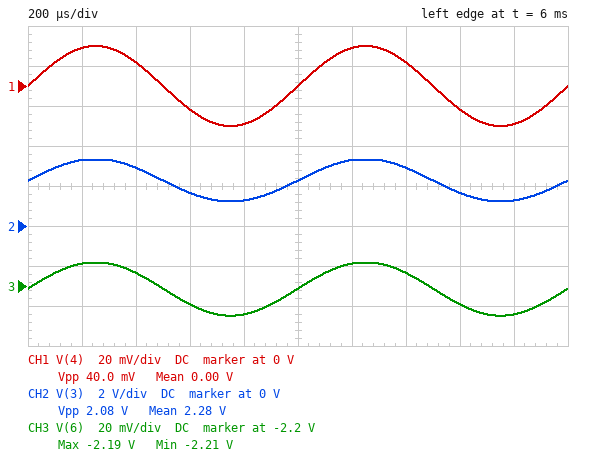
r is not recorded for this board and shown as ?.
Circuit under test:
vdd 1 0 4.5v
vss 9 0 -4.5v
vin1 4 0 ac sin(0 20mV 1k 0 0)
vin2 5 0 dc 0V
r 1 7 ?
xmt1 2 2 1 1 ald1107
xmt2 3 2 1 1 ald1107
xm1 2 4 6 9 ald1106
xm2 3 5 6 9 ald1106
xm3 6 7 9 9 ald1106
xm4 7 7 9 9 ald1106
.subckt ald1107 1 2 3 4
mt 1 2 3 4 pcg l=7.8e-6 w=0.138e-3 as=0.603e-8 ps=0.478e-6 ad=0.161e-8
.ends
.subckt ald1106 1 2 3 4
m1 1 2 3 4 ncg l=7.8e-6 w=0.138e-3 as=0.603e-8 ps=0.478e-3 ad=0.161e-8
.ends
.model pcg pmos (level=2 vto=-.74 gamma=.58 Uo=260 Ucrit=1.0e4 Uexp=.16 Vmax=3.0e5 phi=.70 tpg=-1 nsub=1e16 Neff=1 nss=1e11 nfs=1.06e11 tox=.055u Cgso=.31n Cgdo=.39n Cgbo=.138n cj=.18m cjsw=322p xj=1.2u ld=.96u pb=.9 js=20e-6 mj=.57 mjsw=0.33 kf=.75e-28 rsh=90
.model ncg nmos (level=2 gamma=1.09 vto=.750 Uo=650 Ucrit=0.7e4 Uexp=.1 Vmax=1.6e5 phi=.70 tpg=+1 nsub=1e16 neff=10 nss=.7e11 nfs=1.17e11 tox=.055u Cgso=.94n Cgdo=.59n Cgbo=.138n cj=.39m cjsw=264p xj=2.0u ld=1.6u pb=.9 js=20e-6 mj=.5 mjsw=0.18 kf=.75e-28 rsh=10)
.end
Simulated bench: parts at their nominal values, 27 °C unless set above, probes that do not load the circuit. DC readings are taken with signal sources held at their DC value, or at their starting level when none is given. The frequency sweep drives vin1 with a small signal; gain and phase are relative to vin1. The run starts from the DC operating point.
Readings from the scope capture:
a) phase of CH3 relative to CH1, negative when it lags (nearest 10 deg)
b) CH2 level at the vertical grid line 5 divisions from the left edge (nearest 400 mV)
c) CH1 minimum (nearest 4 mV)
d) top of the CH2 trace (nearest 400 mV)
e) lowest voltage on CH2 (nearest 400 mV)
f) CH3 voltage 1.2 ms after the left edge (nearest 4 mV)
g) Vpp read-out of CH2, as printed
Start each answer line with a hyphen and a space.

- 0 deg
- 2.4 V
- -20 mV
- 3.2 V
- 1.2 V
- -2.188 V
- 2.08 V
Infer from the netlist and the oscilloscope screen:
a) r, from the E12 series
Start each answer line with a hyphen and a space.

- 15 kΩ
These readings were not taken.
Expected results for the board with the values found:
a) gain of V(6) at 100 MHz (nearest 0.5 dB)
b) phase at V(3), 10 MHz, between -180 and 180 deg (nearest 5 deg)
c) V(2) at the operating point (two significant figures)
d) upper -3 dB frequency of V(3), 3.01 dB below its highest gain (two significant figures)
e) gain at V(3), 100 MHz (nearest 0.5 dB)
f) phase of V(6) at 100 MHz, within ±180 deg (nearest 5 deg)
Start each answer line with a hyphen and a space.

- -13.0 dB
- -80 deg
- 2.3 V
- 3.4 MHz
- 0 dB
- -35 deg
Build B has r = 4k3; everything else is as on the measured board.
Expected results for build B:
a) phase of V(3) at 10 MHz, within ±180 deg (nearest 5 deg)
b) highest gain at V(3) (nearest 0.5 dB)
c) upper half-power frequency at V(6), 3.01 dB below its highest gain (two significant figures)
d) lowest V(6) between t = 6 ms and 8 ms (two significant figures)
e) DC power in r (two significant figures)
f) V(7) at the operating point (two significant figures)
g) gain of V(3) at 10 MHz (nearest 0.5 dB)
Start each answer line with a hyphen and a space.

- -60 deg
- 32.0 dB
- 12 MHz
- -2.7 V
- 8.9 mW
- -1.7 V
- 27.5 dB
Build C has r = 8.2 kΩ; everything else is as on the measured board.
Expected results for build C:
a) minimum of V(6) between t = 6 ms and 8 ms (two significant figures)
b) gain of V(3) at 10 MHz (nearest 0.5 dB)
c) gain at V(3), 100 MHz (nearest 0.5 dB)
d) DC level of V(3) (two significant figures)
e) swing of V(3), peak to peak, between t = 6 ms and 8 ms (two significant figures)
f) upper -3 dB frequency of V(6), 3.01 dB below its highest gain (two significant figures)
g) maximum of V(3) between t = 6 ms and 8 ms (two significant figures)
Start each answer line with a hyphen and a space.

- -2.4 V
- 26.0 dB
- 3.5 dB
- 1.8 V
- 1.9 V
- 7.9 MHz
- 2.7 V
